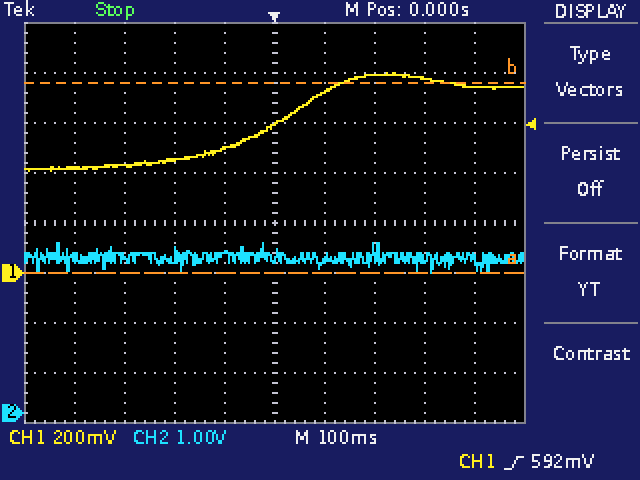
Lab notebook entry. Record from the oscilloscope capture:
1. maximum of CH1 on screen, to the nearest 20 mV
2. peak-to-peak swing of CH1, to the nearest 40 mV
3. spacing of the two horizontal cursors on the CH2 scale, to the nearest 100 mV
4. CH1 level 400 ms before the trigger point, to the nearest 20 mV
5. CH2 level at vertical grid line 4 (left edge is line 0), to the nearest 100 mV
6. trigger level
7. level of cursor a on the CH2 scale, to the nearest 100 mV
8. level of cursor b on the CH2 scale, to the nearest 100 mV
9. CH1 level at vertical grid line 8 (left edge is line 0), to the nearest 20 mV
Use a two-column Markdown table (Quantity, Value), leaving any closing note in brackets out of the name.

| Quantity | Value |
|---|---|
| maximum of CH1 on screen, to the nearest 20 mV | 800 mV |
| peak-to-peak swing of CH1, to the nearest 40 mV | 400 mV |
| spacing of the two horizontal cursors on the CH2 scale, to the nearest 100 mV | 3.8 V |
| CH1 level 400 ms before the trigger point, to the nearest 20 mV | 420 mV |
| CH2 level at vertical grid line 4 (left edge is line 0), to the nearest 100 mV | 3.2 V |
| trigger level | 592 mV |
| level of cursor a on the CH2 scale, to the nearest 100 mV | 2.8 V |
| level of cursor b on the CH2 scale, to the nearest 100 mV | 6.6 V |
| CH1 level at vertical grid line 8 (left edge is line 0), to the nearest 20 mV | 780 mV |
